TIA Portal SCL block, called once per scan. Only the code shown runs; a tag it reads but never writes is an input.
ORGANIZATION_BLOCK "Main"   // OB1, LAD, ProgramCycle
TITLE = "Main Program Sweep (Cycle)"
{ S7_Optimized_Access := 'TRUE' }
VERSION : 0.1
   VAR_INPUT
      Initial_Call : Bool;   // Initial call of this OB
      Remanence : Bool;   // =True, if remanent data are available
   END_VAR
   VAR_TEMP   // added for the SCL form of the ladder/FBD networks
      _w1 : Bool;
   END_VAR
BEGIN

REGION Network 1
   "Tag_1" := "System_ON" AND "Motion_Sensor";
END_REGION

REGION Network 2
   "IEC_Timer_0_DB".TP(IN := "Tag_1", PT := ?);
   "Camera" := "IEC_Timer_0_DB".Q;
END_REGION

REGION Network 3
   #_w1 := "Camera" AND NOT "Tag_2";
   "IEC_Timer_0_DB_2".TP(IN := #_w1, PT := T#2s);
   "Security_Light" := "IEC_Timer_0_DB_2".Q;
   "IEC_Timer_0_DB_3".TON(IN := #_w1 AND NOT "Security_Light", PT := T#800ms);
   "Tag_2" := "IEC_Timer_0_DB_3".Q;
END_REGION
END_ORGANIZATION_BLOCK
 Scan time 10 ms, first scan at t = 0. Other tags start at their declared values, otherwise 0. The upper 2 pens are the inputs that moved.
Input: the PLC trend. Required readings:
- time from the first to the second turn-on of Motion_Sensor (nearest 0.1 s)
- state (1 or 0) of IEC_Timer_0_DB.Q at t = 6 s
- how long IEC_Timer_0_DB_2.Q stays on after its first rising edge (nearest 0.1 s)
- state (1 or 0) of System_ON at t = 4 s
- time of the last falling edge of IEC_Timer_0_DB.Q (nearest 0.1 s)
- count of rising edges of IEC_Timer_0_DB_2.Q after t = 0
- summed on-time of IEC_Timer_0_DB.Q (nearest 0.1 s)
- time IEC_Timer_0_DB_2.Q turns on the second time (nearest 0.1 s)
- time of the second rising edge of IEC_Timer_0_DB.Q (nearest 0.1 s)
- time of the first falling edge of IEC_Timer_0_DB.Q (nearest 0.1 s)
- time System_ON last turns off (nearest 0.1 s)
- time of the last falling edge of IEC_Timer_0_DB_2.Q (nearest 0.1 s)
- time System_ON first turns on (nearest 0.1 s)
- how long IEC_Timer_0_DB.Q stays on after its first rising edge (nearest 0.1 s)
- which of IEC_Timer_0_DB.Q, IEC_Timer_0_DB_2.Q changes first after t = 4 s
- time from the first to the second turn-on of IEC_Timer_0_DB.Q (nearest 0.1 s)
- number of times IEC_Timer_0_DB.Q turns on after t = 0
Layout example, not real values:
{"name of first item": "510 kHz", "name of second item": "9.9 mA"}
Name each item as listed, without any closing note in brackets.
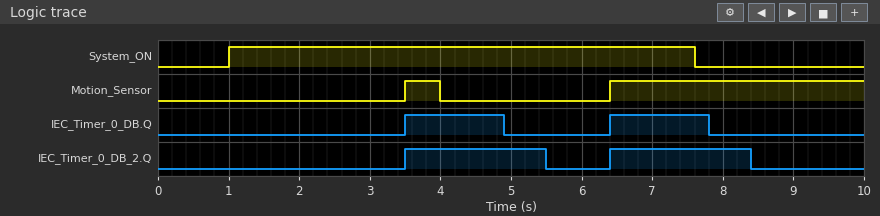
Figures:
{"time from the first to the second turn-on of Motion_Sensor": "2.9 s", "state (1 or 0) of IEC_Timer_0_DB.Q at t = 6 s": "0", "how long IEC_Timer_0_DB_2.Q stays on after its first rising edge": "2.0 s", "state (1 or 0) of System_ON at t = 4 s": "1", "time of the last falling edge of IEC_Timer_0_DB.Q": "7.8 s", "count of rising edges of IEC_Timer_0_DB_2.Q after t = 0": "2", "summed on-time of IEC_Timer_0_DB.Q": "2.8 s", "time IEC_Timer_0_DB_2.Q turns on the second time": "6.4 s", "time of the second rising edge of IEC_Timer_0_DB.Q": "6.4 s", "time of the first falling edge of IEC_Timer_0_DB.Q": "4.9 s", "time System_ON last turns off": "7.6 s", "time of the last falling edge of IEC_Timer_0_DB_2.Q": "8.4 s", "time System_ON first turns on": "1.0 s", "how long IEC_Timer_0_DB.Q stays on after its first rising edge": "1.4 s", "which of IEC_Timer_0_DB.Q, IEC_Timer_0_DB_2.Q changes first after t = 4 s": "IEC_Timer_0_DB.Q", "time from the first to the second turn-on of IEC_Timer_0_DB.Q": "2.9 s", "number of times IEC_Timer_0_DB.Q turns on after t = 0": "2"}
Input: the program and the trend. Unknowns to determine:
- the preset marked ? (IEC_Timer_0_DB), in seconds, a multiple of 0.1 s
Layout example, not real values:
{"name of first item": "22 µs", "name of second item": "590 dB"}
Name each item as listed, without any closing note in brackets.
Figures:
{"the preset marked ? (IEC_Timer_0_DB), in seconds, a multiple of 0.1 s": "1.4 s"}
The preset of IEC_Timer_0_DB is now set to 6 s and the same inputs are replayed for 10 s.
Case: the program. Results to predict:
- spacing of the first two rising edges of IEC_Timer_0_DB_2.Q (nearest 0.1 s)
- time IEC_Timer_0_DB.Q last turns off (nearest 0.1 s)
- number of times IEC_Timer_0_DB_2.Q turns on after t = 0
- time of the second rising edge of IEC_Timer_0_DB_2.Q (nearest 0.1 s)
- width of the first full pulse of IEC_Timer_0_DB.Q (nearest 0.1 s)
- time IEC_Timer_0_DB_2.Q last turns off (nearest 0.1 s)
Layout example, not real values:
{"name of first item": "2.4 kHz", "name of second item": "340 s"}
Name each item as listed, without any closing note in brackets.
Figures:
{"spacing of the first two rising edges of IEC_Timer_0_DB_2.Q": "2.8 s", "time IEC_Timer_0_DB.Q last turns off": "9.5 s", "number of times IEC_Timer_0_DB_2.Q turns on after t = 0": "3", "time of the second rising edge of IEC_Timer_0_DB_2.Q": "6.3 s", "width of the first full pulse of IEC_Timer_0_DB.Q": "6.0 s", "time IEC_Timer_0_DB_2.Q last turns off": "8.3 s"}
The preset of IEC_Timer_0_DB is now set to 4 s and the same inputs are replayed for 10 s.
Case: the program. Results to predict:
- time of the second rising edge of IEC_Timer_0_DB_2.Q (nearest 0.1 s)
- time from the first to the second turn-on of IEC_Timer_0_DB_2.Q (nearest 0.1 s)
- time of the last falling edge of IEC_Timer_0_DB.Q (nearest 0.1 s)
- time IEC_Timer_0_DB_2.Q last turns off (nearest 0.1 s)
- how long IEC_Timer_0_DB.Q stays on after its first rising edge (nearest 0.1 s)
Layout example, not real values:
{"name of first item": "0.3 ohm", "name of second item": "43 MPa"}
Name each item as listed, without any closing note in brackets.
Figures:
{"time of the second rising edge of IEC_Timer_0_DB_2.Q": "6.3 s", "time from the first to the second turn-on of IEC_Timer_0_DB_2.Q": "2.8 s", "time of the last falling edge of IEC_Timer_0_DB.Q": "7.5 s", "time IEC_Timer_0_DB_2.Q last turns off": "8.3 s", "how long IEC_Timer_0_DB.Q stays on after its first rising edge": "4.0 s"}
